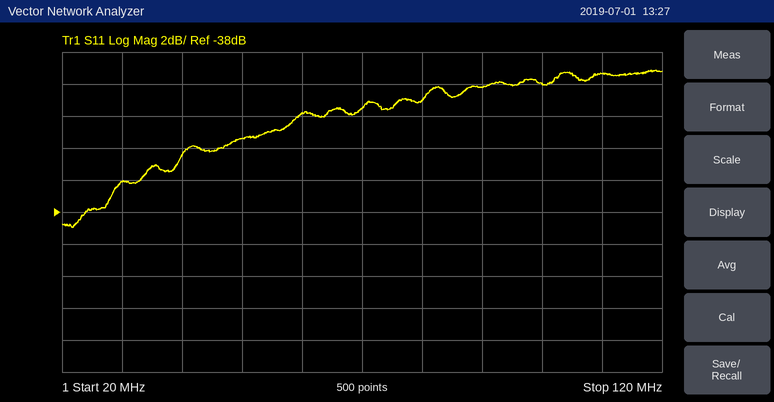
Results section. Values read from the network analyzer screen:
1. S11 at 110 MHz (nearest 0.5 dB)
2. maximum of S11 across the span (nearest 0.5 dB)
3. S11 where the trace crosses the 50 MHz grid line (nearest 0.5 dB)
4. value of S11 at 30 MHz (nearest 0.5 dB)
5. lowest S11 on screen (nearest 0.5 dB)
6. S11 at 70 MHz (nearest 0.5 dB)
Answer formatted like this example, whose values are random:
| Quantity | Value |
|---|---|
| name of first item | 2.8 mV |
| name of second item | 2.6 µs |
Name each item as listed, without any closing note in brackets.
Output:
| Quantity | Value |
|---|---|
| S11 at 110 MHz | -29.5 dB |
| maximum of S11 across the span | -29.0 dB |
| S11 where the trace crosses the 50 MHz grid line | -33.5 dB |
| value of S11 at 30 MHz | -36.0 dB |
| lowest S11 on screen | -39.0 dB |
| S11 at 70 MHz | -31.5 dB |
